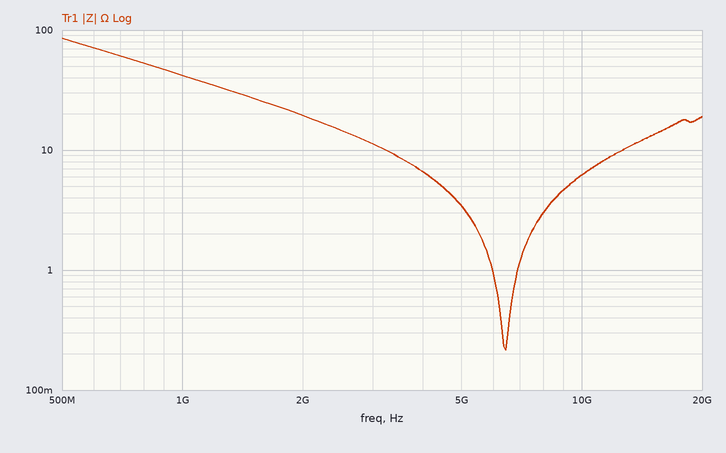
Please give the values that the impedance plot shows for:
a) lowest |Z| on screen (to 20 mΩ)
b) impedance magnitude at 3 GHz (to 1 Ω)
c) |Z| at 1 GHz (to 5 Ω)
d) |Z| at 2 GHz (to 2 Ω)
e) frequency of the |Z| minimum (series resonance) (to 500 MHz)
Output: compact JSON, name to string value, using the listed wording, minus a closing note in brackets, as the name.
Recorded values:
{"lowest |Z| on screen": "220 mΩ", "impedance magnitude at 3 GHz": "11 Ω", "|Z| at 1 GHz": "40 Ω", "|Z| at 2 GHz": "20 Ω", "frequency of the |Z| minimum (series resonance)": "6.5 GHz"}
